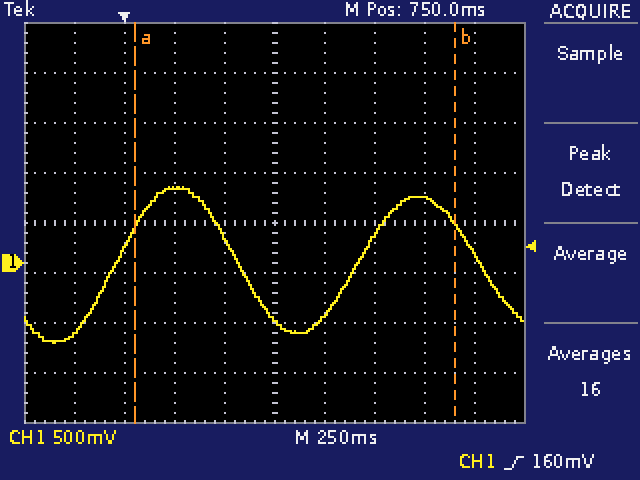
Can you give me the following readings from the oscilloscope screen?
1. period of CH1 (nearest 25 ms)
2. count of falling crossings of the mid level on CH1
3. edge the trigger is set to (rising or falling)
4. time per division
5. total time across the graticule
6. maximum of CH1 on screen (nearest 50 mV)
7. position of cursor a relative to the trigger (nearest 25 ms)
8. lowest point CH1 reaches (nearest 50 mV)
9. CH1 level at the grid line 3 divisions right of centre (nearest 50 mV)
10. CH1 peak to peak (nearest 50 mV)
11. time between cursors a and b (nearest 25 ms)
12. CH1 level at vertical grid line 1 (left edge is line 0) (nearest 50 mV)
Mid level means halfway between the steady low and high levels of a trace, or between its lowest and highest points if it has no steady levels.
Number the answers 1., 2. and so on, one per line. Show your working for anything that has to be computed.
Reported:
1. 1.200 s
2. 2
3. rising
4. 250 ms
5. 2.5 s
6. 750 mV
7. +50 ms
8. -800 mV
9. 650 mV
10. 750 mV − (-800 mV) = 1.55 V
11. 1.600 s
12. -700 mV
